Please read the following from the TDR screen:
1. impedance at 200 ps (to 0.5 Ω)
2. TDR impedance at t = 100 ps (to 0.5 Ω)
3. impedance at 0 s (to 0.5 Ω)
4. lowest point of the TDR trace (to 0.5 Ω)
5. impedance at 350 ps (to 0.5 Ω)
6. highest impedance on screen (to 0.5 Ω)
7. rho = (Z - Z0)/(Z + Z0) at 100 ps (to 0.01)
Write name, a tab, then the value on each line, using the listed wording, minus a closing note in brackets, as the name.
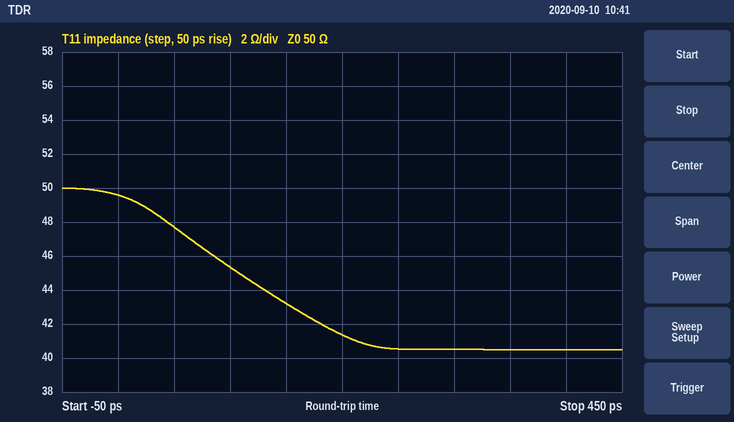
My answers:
impedance at 200 ps	41.5 Ω
TDR impedance at t = 100 ps	45.5 Ω
impedance at 0 s	49.5 Ω
lowest point of the TDR trace	40.5 Ω
impedance at 350 ps	40.5 Ω
highest impedance on screen	50.0 Ω
rho = (Z - Z0)/(Z + Z0) at 100 ps	-0.05
